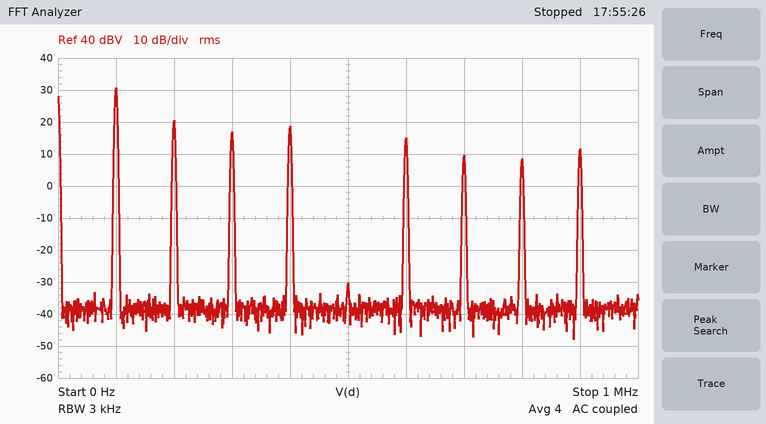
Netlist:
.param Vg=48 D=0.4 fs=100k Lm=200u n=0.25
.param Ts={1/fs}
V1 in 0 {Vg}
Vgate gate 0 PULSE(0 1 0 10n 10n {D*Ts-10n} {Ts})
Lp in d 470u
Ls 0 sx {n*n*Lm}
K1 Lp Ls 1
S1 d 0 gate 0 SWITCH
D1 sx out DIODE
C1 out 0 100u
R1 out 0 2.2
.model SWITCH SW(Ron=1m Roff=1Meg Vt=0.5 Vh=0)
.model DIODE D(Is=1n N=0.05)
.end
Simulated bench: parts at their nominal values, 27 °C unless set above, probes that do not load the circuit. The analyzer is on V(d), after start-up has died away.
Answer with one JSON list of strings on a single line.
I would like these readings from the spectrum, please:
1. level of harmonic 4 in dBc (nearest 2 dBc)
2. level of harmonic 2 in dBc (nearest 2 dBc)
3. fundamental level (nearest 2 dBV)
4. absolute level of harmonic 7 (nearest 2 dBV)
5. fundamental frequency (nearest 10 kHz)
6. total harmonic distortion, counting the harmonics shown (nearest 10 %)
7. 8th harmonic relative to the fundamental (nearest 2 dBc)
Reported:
["-12 dBc", "-10 dBc", "30 dBV", "10 dBV", "100 kHz", "50 %", "-22 dBc"]
